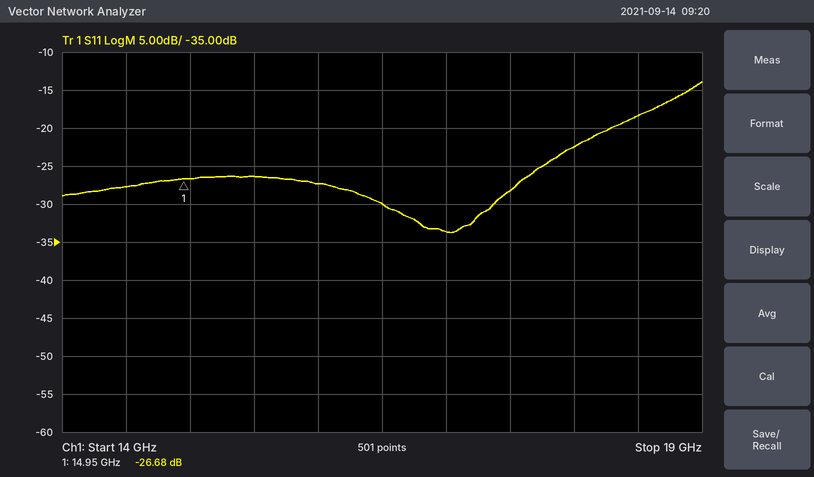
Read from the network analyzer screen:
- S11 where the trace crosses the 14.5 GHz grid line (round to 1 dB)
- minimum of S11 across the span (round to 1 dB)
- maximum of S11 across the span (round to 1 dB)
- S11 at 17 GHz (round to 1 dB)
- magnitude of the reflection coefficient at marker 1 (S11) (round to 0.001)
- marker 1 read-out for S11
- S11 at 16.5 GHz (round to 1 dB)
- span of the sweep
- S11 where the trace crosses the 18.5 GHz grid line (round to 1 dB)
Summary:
-28 dB
-34 dB
-14 dB
-34 dB
0.046
-26.68 dB
-30 dB
5 GHz
-18 dB
